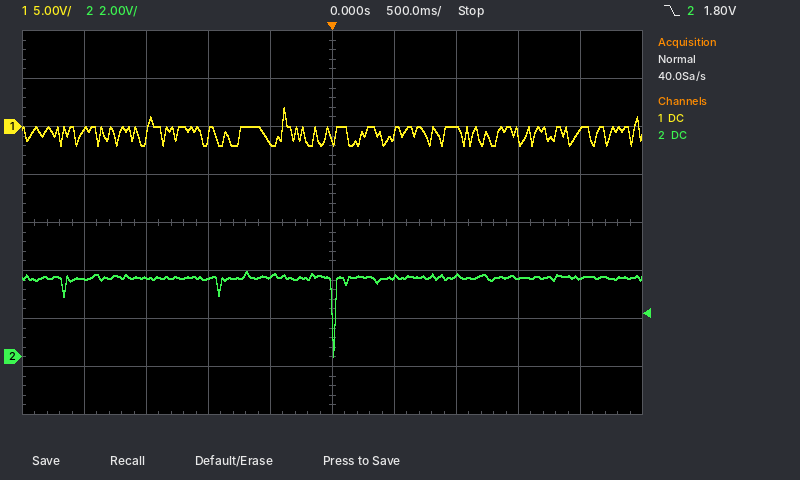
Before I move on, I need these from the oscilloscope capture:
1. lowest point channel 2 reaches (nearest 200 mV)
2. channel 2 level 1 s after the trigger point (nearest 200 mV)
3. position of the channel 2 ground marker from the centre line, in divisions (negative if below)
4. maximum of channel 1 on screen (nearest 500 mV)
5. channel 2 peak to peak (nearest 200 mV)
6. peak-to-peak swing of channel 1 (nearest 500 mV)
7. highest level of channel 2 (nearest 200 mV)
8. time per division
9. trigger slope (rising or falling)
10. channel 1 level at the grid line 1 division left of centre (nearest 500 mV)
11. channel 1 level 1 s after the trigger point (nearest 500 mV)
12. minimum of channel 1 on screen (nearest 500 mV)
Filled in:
0.0 V
3.4 V
-2.8 div
2.0 V
3.6 V
4.0 V
3.6 V
500 ms
falling
-1.5 V
0.0 V
-2.0 V
